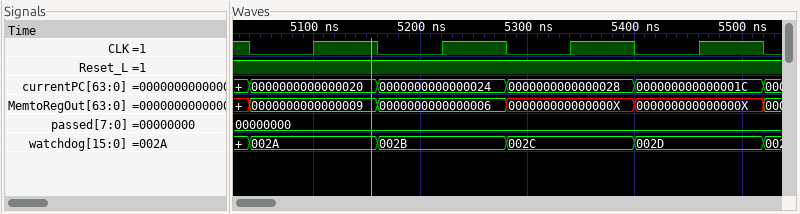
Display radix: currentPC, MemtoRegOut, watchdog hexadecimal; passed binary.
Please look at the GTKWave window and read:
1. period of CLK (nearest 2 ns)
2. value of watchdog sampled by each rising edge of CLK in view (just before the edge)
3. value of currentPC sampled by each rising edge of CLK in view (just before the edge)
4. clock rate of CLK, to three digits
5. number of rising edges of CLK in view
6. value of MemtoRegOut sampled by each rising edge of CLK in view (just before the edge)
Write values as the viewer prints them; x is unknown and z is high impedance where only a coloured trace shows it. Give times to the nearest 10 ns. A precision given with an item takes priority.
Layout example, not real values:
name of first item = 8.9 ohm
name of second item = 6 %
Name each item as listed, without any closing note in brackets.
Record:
period of CLK = 120 ns
value of watchdog sampled by each rising edge of CLK in view = 002A, 002B, 002C, 002D
value of currentPC sampled by each rising edge of CLK in view = 0000000000000020, 0000000000000024, 0000000000000028, 000000000000001C
clock rate of CLK, to three digits = 8.33 MHz
number of rising edges of CLK in view = 4
value of MemtoRegOut sampled by each rising edge of CLK in view = 0000000000000009, 0000000000000006, 000000000000000X, 000000000000000X
